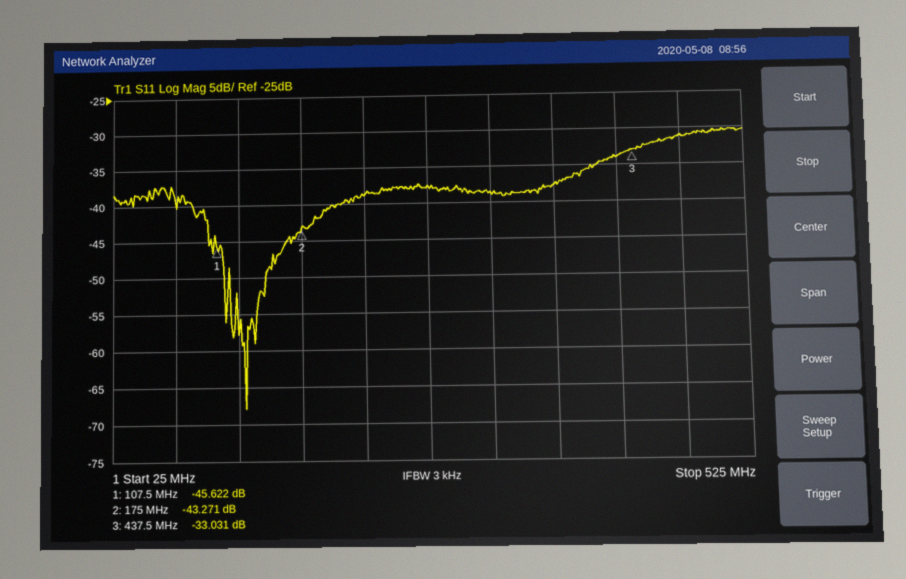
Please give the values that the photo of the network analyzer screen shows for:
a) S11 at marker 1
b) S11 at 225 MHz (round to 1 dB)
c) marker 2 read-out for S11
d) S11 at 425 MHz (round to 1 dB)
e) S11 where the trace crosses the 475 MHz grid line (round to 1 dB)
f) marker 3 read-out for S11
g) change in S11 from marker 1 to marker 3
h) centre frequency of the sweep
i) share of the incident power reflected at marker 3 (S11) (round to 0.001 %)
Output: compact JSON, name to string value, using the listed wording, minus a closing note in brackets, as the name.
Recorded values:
{"S11 at marker 1": "-45.622 dB", "S11 at 225 MHz": "-39 dB", "marker 2 read-out for S11": "-43.271 dB", "S11 at 425 MHz": "-34 dB", "S11 where the trace crosses the 475 MHz grid line": "-31 dB", "marker 3 read-out for S11": "-33.031 dB", "change in S11 from marker 1 to marker 3": "12.591 dB", "centre frequency of the sweep": "275 MHz", "share of the incident power reflected at marker 3 (S11)": "0.050 %"}
